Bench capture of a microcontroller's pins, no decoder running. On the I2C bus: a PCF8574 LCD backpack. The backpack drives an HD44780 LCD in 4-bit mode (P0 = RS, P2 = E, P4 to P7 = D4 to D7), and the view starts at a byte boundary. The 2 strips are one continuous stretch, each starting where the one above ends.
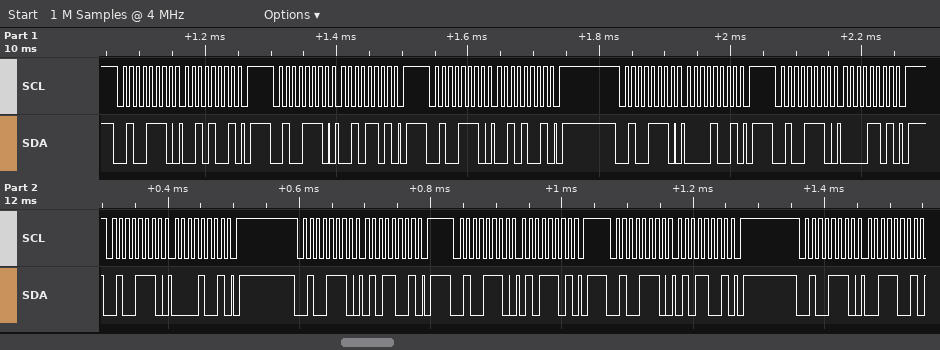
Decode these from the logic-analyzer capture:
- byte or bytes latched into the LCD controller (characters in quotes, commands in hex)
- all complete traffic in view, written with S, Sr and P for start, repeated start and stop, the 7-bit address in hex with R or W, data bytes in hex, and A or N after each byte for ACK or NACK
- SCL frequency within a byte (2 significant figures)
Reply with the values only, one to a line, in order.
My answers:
' '
S 27W A 29 A P S 27W A 2D A P S 27W A 29 A P S 27W A 09 A P S 27W A 0D A P S 27W A 09 A P S 27W A 59 A P S 27W A 5D A P S 27W A 59 A P S 27W A 39 A
100 kHz
